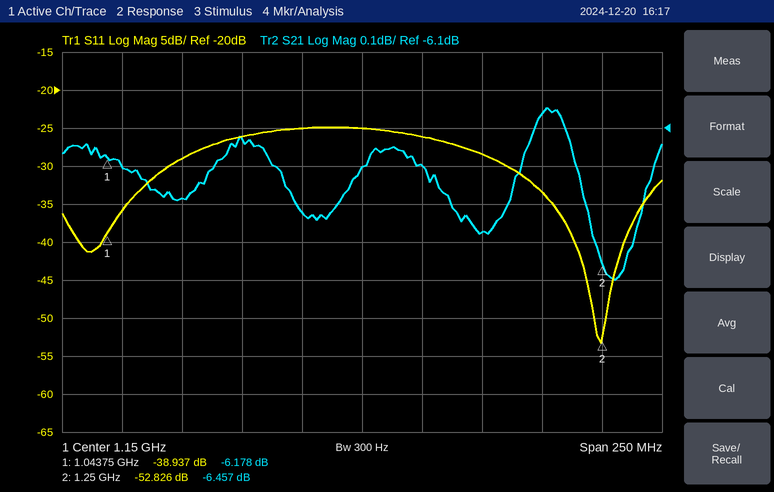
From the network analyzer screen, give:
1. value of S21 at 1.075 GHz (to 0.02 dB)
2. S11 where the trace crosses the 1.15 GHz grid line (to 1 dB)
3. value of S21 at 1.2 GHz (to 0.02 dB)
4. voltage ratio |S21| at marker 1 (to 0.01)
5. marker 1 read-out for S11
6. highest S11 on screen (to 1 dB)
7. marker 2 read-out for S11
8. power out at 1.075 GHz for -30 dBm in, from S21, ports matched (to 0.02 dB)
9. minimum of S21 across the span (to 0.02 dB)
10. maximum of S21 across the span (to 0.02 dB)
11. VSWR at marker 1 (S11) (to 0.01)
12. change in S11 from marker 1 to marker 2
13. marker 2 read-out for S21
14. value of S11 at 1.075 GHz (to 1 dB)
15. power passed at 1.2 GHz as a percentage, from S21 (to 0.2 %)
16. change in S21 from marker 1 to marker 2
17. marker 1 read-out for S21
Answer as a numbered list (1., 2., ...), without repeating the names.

1. -6.28 dB
2. -25 dB
3. -6.38 dB
4. 0.49
5. -38.937 dB
6. -25 dB
7. -52.826 dB
8. -36.28 dBm
9. -6.50 dB
10. -6.04 dB
11. 1.02
12. -13.889 dB
13. -6.457 dB
14. -29 dB
15. 23.0 %
16. -0.279 dB
17. -6.178 dB
